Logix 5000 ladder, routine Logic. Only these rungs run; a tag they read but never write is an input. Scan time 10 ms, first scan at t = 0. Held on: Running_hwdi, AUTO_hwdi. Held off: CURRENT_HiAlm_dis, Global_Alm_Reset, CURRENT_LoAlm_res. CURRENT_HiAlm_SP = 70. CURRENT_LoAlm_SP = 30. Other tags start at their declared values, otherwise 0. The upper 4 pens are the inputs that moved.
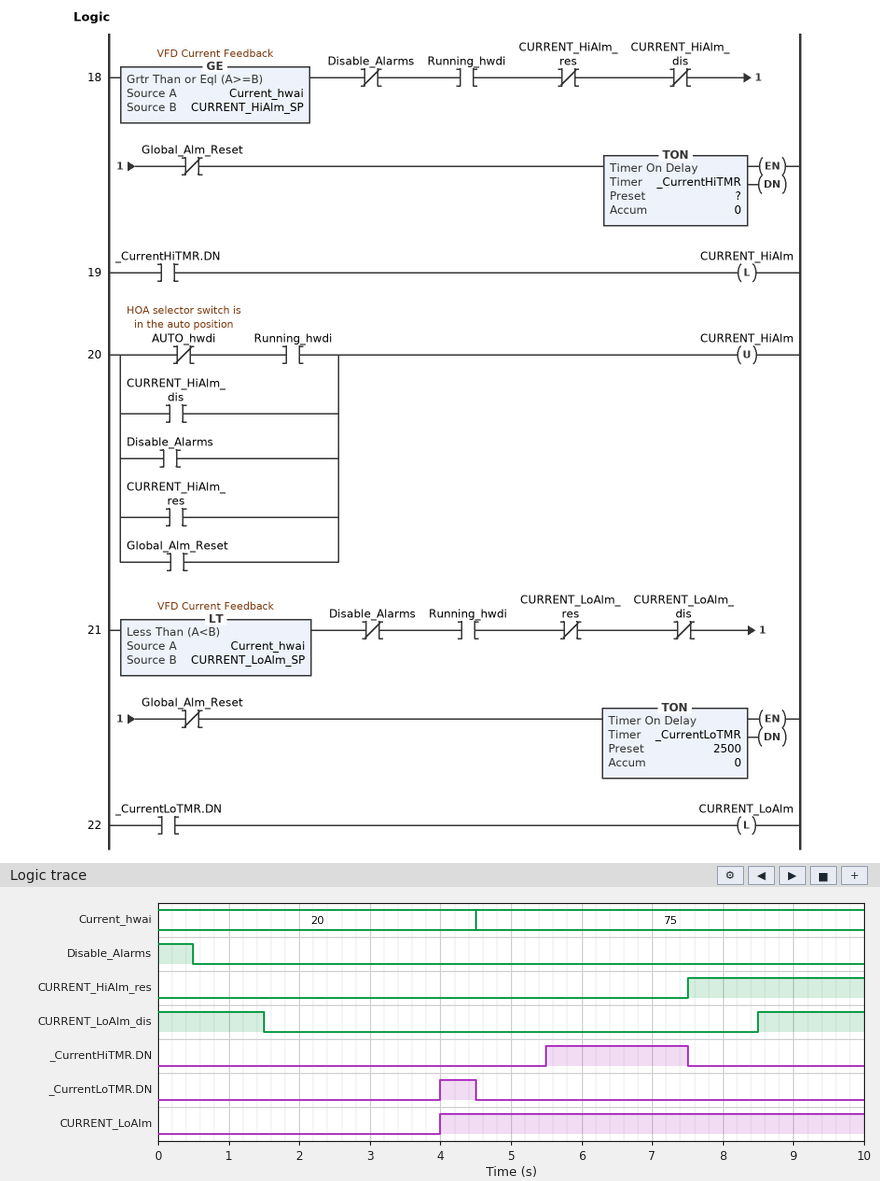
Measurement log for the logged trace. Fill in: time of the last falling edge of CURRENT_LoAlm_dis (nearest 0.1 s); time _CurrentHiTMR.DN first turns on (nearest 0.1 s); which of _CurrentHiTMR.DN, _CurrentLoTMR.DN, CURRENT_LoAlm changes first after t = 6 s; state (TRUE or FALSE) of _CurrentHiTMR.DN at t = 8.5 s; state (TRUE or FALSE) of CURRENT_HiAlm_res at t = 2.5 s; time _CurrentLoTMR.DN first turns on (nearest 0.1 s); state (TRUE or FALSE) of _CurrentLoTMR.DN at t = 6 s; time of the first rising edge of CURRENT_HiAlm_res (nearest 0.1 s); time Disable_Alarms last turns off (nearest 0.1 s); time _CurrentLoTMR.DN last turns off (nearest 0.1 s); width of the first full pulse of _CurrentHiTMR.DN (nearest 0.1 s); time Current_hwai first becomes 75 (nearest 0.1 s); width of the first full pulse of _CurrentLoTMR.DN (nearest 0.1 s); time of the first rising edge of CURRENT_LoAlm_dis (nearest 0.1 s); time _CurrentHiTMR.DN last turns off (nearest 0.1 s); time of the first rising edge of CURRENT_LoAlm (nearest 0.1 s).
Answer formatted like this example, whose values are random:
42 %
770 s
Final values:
1.5 s
5.5 s
_CurrentHiTMR.DN
FALSE
FALSE
4.0 s
FALSE
7.5 s
0.5 s
4.5 s
2.0 s
4.5 s
0.5 s
8.5 s
7.5 s
4.0 s
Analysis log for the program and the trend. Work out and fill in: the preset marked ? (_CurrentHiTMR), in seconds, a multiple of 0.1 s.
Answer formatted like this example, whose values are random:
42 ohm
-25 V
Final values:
1.0 s
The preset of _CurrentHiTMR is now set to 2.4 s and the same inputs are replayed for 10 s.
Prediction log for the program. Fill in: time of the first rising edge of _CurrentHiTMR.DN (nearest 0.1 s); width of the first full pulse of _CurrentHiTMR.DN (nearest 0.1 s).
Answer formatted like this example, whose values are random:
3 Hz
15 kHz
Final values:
6.9 s
0.6 s
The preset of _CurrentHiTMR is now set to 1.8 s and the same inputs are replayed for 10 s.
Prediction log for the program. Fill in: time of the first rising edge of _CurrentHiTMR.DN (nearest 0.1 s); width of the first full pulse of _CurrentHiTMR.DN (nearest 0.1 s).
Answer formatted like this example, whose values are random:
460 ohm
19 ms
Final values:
6.3 s
1.2 s
